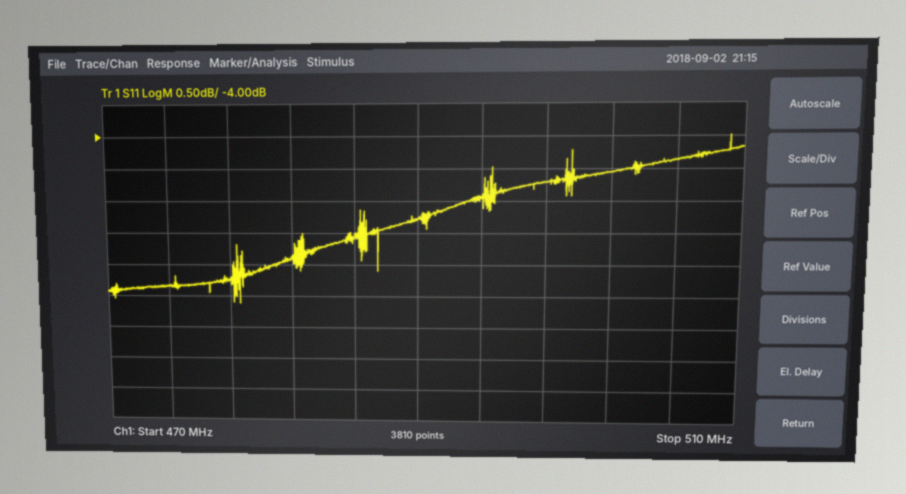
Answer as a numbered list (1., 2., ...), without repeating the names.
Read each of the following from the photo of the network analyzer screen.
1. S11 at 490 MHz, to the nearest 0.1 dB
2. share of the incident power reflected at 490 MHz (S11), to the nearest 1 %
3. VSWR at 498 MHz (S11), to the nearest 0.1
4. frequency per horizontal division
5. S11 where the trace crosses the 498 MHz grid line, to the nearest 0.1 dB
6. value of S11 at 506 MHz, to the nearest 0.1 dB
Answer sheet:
1. -5.3 dB
2. 30 %
3. 3.8
4. 4 MHz
5. -4.7 dB
6. -4.4 dB
